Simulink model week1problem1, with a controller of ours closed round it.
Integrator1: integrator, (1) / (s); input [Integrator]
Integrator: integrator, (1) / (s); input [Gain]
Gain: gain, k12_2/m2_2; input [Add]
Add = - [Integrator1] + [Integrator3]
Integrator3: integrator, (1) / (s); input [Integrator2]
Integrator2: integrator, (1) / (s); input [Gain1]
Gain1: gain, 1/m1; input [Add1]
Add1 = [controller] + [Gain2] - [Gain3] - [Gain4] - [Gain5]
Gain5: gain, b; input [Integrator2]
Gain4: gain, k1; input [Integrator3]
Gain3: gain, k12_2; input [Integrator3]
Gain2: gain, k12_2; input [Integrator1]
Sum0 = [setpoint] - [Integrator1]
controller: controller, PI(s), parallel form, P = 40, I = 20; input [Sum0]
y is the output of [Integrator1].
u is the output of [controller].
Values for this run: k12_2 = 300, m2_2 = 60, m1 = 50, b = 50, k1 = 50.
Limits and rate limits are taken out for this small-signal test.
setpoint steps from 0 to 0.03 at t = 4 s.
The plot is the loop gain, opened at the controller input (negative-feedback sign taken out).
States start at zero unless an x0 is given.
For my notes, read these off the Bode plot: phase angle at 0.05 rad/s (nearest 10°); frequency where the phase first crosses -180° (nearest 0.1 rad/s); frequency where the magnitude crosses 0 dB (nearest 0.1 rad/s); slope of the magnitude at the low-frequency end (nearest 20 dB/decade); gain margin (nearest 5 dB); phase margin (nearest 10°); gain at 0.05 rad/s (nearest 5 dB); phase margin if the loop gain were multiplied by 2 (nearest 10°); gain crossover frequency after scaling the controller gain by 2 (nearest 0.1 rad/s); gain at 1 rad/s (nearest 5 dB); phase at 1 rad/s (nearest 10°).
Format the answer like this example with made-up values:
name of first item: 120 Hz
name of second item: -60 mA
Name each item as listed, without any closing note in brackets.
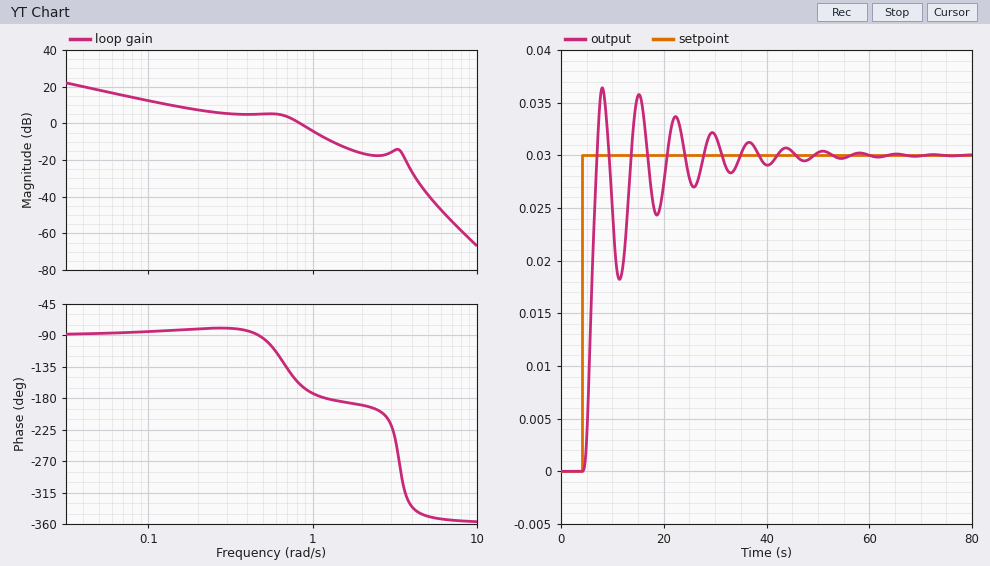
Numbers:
phase angle at 0.05 rad/s: -90°
frequency where the phase first crosses -180°: 1.2 rad/s
frequency where the magnitude crosses 0 dB: 0.8 rad/s
slope of the magnitude at the low-frequency end: -20 dB/decade
gain margin: 10 dB
phase margin: 20°
gain at 0.05 rad/s: 20 dB
phase margin if the loop gain were multiplied by 2: 0°
gain crossover frequency after scaling the controller gain by 2: 1.1 rad/s
gain at 1 rad/s: -5 dB
phase at 1 rad/s: -170°
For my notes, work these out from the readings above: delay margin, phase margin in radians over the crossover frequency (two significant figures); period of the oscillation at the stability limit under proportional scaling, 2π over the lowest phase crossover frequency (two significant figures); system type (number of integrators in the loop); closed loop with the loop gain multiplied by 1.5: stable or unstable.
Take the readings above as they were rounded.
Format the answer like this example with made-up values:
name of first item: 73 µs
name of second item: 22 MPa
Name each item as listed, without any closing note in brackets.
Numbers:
delay margin, phase margin in radians over the crossover frequency: 0.44 s
period of the oscillation at the stability limit under proportional scaling, 2π over the lowest phase crossover frequency: 5.2 s
system type: 1
closed loop with the loop gain multiplied by 1.5: stable or unstable: stable
